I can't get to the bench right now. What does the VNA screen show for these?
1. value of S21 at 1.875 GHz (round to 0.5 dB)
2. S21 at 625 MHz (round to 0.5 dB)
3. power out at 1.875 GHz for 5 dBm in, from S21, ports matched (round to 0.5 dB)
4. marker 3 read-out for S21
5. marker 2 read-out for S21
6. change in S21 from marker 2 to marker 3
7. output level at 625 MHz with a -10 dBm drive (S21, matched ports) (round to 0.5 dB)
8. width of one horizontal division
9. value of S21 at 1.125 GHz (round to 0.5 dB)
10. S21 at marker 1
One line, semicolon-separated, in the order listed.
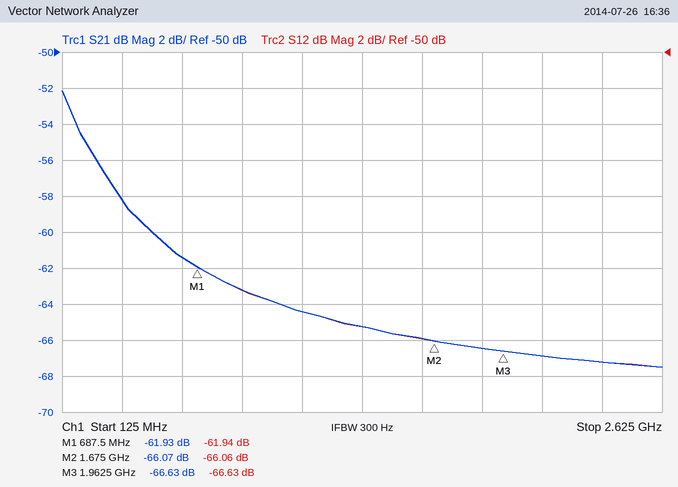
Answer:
-66.5 dB; -61.5 dB; -61.5 dBm; -66.63 dB; -66.07 dB; -0.56 dB; -71.5 dBm; 250 MHz; -64.5 dB; -61.93 dB
